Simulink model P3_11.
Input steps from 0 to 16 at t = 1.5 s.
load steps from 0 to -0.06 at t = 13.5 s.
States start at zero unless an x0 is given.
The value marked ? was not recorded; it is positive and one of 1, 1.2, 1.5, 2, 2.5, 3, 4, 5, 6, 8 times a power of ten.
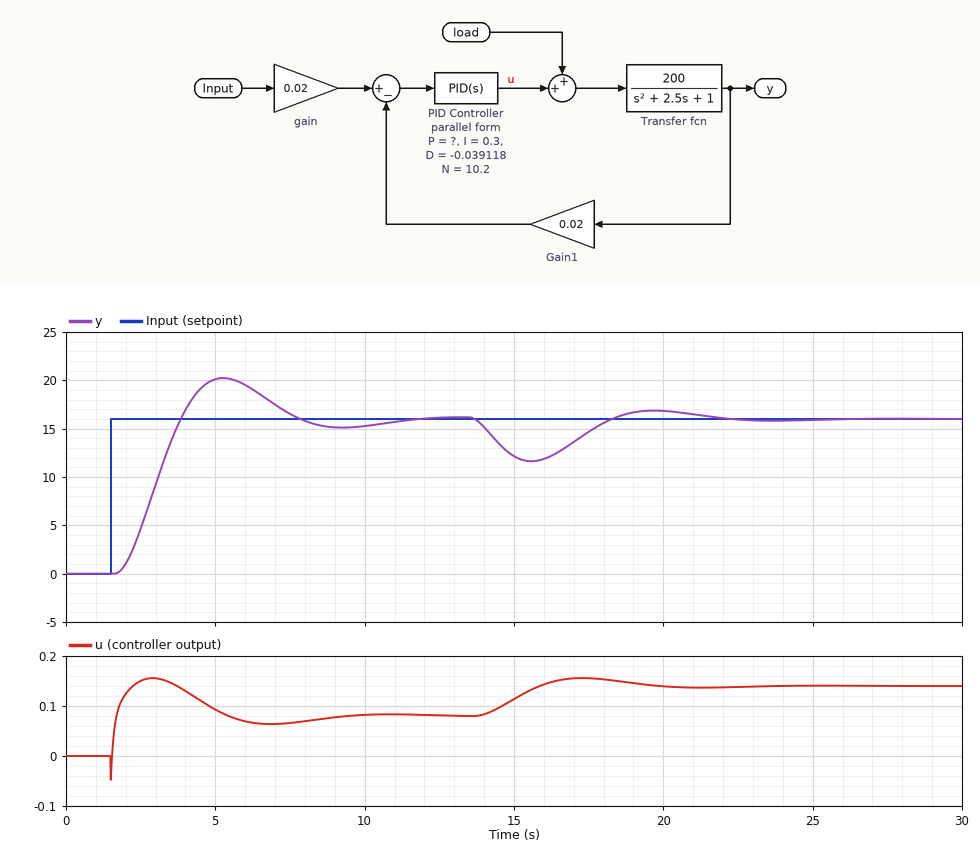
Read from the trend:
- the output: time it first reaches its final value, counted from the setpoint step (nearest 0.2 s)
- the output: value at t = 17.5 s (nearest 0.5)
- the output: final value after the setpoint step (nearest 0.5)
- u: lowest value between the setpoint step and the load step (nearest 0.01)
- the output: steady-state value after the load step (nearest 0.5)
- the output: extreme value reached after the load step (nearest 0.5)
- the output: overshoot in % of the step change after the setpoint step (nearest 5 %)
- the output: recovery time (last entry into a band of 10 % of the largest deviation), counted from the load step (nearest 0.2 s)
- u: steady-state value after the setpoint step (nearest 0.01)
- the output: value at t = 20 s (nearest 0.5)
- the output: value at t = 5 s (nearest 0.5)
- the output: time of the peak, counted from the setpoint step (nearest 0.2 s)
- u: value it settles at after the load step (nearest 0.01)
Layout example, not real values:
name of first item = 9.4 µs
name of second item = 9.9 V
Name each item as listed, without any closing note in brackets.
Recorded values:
the output: time it first reaches its final value, counted from the setpoint step = 2.4 s
the output: value at t = 17.5 s = 14.5
the output: final value after the setpoint step = 16.0
u: lowest value between the setpoint step and the load step = -0.05
the output: steady-state value after the load step = 16.0
the output: extreme value reached after the load step = 11.5
the output: overshoot in % of the step change after the setpoint step = 25 %
the output: recovery time (last entry into a band of 10 % of the largest deviation), counted from the load step = 7.6 s
u: steady-state value after the setpoint step = 0.08
the output: value at t = 20 s = 17.0
the output: value at t = 5 s = 20.0
the output: time of the peak, counted from the setpoint step = 3.8 s
u: value it settles at after the load step = 0.14
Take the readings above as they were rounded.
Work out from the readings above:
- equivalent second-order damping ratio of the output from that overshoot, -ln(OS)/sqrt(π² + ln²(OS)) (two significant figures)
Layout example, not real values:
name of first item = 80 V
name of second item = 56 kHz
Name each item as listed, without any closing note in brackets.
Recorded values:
equivalent second-order damping ratio of the output from that overshoot, -ln(OS)/sqrt(π² + ln²(OS)) = 0.40
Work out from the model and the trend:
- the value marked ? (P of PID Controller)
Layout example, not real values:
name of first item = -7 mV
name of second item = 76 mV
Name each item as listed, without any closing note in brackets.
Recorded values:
the value marked ? = 0.25
